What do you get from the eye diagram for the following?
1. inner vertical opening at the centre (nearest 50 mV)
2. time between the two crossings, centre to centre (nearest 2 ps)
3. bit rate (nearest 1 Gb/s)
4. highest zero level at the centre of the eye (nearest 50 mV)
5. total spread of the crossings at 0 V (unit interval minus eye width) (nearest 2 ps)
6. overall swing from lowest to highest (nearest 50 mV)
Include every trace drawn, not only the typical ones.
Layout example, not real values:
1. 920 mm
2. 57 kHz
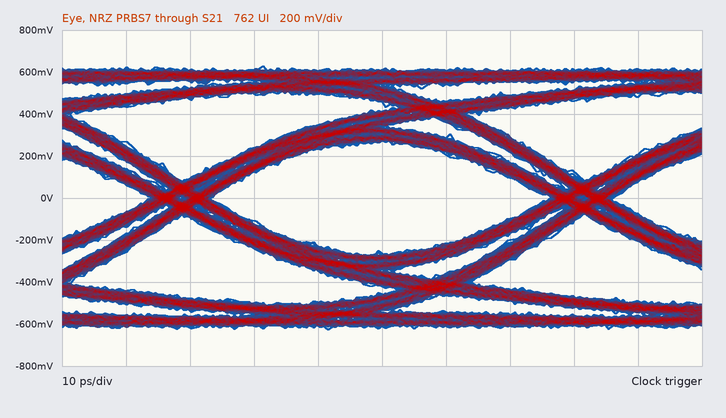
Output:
1. 550 mV
2. 62 ps
3. 16 Gb/s
4. -250 mV
5. 10 ps
6. 1.25 V
